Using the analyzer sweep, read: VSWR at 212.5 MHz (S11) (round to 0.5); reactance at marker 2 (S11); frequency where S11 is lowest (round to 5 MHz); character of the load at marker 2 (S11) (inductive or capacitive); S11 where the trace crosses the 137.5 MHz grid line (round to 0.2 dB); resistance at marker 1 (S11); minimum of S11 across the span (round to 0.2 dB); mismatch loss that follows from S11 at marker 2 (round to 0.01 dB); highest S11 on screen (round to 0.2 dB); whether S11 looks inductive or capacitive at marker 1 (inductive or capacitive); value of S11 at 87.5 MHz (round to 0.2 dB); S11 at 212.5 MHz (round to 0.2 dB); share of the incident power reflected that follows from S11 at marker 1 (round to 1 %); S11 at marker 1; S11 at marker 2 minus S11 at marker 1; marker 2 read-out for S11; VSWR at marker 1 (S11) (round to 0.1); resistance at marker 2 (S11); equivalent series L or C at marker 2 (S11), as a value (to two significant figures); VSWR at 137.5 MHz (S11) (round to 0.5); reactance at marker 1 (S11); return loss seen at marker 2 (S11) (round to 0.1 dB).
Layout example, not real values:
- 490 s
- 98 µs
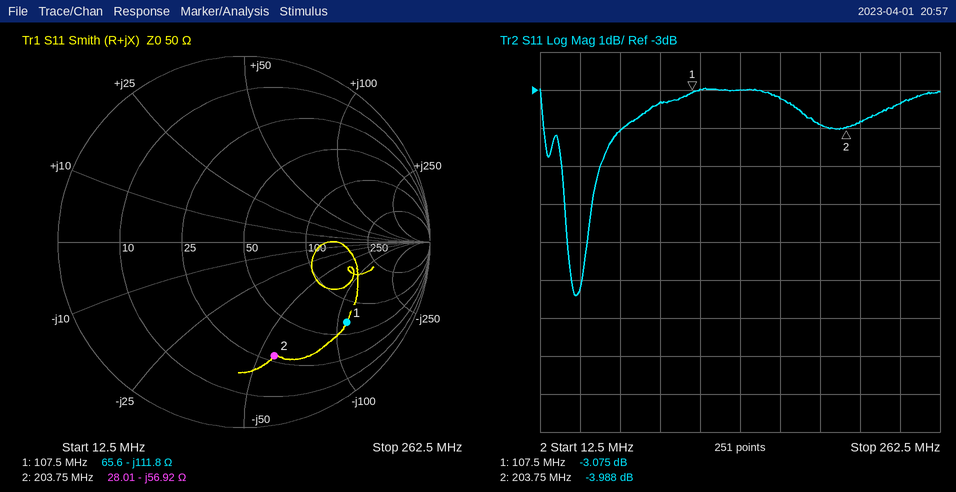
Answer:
- 4.5
- -56.92 Ω
- 35 MHz
- capacitive
- -3.0 dB
- 65.6 Ω
- -8.4 dB
- 2.21 dB
- -3.0 dB
- capacitive
- -3.4 dB
- -3.8 dB
- 49 %
- -3.075 dB
- -0.913 dB
- -3.988 dB
- 5.7
- 28.01 Ω
- 14 pF
- 6.0
- -111.8 Ω
- 4.0 dB
